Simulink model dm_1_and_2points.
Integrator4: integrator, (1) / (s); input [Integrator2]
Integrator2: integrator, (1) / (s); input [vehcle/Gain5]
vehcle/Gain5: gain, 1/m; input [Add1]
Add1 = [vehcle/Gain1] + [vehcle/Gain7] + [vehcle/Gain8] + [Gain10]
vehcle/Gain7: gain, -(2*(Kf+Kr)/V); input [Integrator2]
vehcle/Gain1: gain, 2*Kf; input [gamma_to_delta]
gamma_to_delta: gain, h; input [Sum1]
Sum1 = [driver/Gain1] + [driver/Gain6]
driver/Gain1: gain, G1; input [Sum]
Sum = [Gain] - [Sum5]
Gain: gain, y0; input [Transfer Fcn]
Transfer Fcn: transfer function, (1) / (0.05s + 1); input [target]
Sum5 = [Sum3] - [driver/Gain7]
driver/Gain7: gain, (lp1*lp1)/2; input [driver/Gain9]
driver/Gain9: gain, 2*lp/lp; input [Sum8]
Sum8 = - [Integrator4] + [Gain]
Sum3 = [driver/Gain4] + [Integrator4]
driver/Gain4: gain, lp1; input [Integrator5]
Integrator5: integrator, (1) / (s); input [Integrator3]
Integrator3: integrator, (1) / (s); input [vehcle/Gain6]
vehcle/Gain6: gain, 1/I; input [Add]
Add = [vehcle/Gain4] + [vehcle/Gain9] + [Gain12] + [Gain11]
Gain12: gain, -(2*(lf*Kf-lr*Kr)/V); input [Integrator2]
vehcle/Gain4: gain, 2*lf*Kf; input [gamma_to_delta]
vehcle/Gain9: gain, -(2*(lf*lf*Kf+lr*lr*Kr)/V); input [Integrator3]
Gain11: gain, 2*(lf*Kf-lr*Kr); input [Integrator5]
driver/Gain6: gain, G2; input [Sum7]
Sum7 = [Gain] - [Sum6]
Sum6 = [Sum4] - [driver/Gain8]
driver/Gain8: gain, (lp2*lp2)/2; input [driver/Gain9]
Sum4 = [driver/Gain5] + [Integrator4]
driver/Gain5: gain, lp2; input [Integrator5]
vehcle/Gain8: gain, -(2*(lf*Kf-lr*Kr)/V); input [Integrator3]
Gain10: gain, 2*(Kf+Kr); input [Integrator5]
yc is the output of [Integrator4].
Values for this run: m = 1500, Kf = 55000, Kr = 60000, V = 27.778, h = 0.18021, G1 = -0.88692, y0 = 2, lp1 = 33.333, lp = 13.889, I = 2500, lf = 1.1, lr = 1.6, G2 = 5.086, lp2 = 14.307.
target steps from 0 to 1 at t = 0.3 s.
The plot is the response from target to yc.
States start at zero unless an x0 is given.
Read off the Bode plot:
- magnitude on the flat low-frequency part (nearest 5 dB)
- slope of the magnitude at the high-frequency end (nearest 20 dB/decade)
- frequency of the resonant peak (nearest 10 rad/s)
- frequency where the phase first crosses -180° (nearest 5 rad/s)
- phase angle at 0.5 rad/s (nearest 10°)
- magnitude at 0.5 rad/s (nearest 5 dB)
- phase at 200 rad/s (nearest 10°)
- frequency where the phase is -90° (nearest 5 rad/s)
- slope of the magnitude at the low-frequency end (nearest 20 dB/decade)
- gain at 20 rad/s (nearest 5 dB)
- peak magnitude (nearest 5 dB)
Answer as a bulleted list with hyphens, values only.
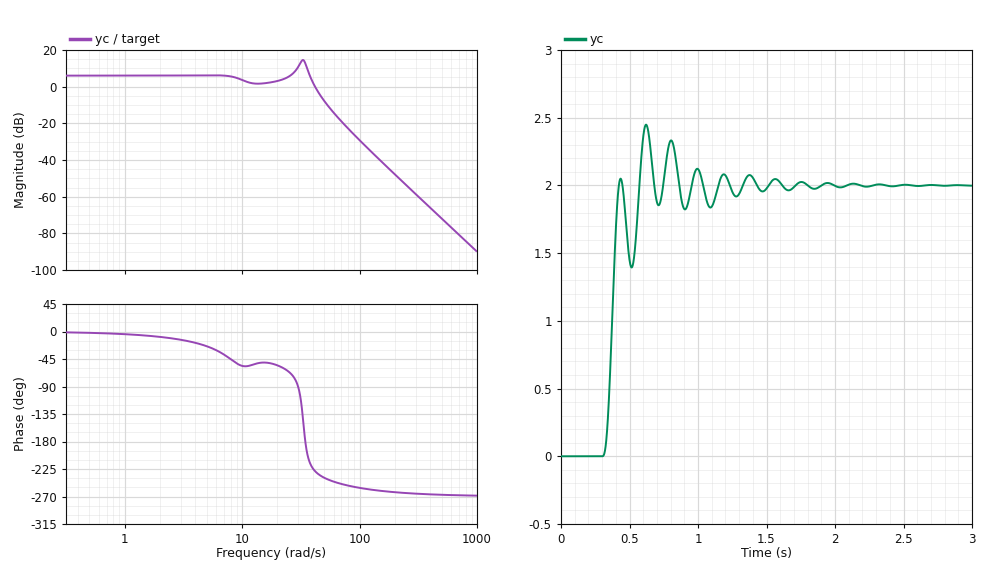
- 5 dB
- -60 dB/decade
- 30 rad/s
- 35 rad/s
- 0°
- 5 dB
- -260°
- 30 rad/s
- 0 dB/decade
- 5 dB
- 15 dB
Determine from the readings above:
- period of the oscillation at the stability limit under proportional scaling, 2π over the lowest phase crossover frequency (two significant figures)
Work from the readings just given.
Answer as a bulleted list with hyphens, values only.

- 0.18 s
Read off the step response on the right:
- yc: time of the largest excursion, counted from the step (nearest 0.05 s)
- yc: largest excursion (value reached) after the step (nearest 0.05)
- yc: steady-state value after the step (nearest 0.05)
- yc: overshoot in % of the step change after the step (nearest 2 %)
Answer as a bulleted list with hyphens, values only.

- 0.30 s
- 2.45
- 2.00
- 22 %
